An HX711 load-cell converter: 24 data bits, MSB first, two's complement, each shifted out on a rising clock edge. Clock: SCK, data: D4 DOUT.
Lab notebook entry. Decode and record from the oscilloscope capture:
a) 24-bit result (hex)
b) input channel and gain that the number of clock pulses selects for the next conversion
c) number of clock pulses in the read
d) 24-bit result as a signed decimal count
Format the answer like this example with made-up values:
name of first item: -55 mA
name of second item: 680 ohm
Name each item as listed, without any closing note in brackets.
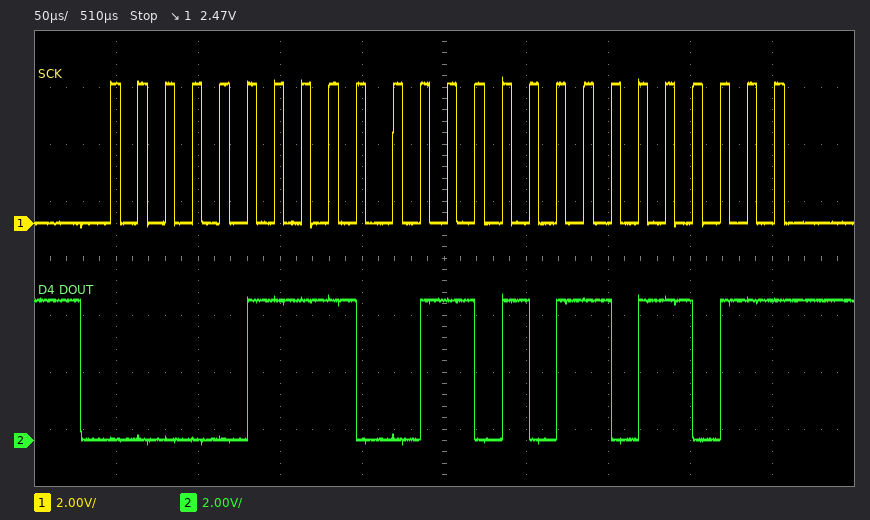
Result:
24-bit result: 0x079ADB
input channel and gain that the number of clock pulses selects for the next conversion: channel A, gain 128
number of clock pulses in the read: 25
24-bit result as a signed decimal count: 498395
